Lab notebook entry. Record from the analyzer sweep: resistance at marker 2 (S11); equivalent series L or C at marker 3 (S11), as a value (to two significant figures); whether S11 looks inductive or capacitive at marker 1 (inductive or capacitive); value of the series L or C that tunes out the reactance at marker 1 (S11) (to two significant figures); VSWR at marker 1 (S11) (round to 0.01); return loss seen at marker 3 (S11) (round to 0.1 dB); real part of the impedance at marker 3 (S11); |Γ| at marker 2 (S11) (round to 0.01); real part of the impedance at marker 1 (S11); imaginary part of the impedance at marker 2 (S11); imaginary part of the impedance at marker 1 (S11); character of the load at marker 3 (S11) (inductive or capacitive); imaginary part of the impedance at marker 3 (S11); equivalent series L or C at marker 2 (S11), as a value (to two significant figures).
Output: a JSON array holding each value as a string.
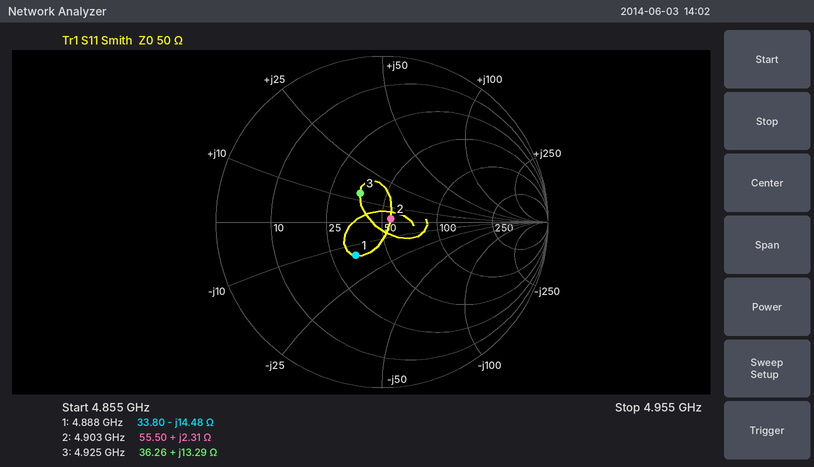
["55.50 Ω", "430 pH", "capacitive", "470 pH", "1.69", "13.2 dB", "36.26 Ω", "0.06", "33.80 Ω", "+2.31 Ω", "-14.48 Ω", "inductive", "+13.29 Ω", "75 pH"]
